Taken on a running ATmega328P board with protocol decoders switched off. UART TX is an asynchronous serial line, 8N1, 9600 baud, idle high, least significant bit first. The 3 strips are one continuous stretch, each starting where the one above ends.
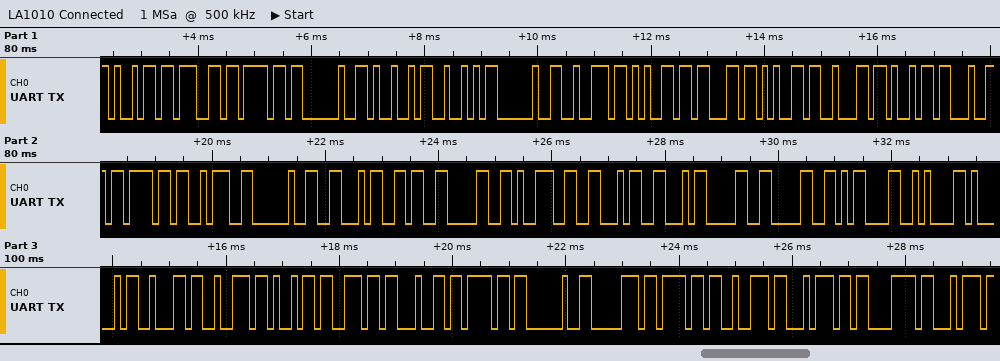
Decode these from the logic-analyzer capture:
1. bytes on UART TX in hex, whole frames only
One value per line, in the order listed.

69 67 6F 20 49 52 20 72 65 63 65 62 69 64 6F 3A 20 46 36 30 39 46 46 30 30 0D 0A 41 62 72 69 6E 64 6F 20 70 6F 72 74 C3 A3
